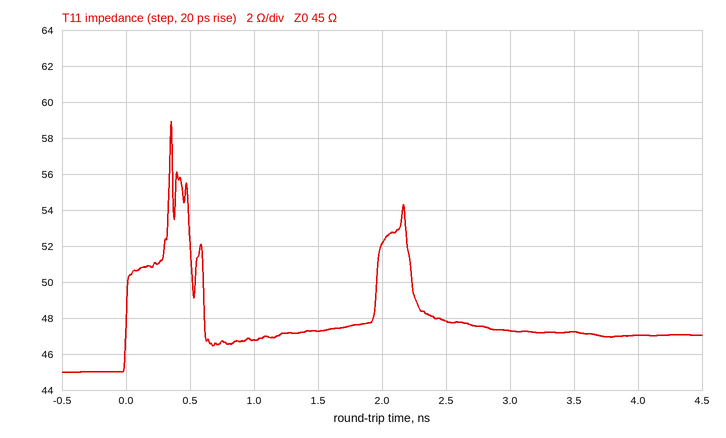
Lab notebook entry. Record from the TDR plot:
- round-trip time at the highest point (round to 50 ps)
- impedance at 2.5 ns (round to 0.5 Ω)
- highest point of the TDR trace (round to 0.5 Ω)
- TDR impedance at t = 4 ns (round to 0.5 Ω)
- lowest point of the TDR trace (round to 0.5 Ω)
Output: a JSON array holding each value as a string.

["350 ps", "48.0 Ω", "59.0 Ω", "47.0 Ω", "45.0 Ω"]
